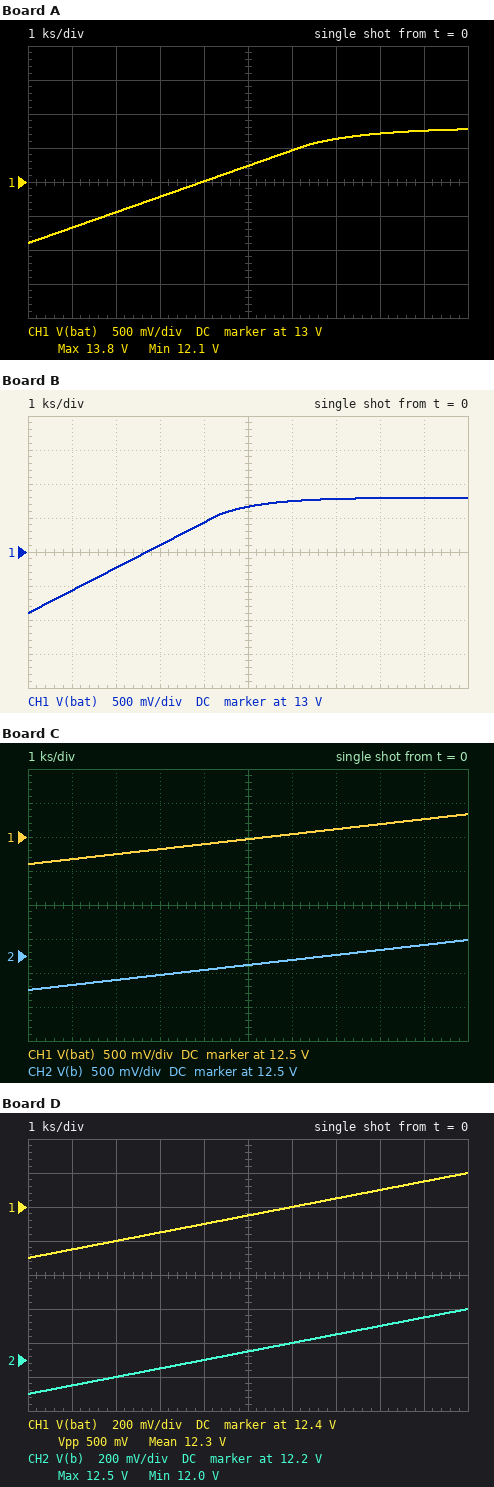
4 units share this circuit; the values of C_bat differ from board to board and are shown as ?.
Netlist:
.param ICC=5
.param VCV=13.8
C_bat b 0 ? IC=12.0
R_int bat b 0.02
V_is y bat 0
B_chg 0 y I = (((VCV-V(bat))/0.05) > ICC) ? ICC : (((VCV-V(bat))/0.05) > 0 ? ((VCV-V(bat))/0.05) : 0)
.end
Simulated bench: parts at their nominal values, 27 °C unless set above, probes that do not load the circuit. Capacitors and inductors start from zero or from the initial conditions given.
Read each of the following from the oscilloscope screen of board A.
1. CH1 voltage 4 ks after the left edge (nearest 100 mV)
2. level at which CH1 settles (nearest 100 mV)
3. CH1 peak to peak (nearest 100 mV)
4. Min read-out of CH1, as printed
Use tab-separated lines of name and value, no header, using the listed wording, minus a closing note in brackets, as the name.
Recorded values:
CH1 voltage 4 ks after the left edge	13.0 V
level at which CH1 settles	13.8 V
CH1 peak to peak	1.7 V
Min read-out of CH1, as printed	12.1 V
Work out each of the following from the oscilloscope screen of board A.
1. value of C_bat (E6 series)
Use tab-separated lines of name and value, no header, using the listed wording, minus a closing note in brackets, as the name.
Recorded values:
value of C_bat	22 kF
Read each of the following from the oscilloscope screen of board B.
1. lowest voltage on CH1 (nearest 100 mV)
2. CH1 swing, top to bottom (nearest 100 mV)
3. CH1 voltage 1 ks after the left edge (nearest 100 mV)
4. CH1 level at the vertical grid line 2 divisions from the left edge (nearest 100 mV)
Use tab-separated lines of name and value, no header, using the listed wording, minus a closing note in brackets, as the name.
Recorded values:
lowest voltage on CH1	12.1 V
CH1 swing, top to bottom	1.7 V
CH1 voltage 1 ks after the left edge	12.4 V
CH1 level at the vertical grid line 2 divisions from the left edge	12.8 V
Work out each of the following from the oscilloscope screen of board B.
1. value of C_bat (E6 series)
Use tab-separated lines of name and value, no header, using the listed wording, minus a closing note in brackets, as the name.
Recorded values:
value of C_bat	15 kF
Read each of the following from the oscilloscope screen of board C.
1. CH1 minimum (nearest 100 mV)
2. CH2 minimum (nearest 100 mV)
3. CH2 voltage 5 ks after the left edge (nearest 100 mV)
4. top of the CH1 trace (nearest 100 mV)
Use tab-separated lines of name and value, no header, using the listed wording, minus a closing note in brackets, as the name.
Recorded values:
CH1 minimum	12.1 V
CH2 minimum	12.0 V
CH2 voltage 5 ks after the left edge	12.4 V
top of the CH1 trace	12.8 V
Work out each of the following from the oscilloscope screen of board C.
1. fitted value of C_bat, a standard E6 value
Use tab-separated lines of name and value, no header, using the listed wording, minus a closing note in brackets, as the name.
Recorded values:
fitted value of C_bat, a standard E6 value	68 kF
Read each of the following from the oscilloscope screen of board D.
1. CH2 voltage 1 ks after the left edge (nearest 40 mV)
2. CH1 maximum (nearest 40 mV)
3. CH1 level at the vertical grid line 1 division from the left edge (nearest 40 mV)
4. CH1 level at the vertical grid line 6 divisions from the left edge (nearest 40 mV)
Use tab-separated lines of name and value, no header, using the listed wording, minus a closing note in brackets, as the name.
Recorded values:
CH2 voltage 1 ks after the left edge	12.04 V
CH1 maximum	12.60 V
CH1 level at the vertical grid line 1 division from the left edge	12.16 V
CH1 level at the vertical grid line 6 divisions from the left edge	12.40 V
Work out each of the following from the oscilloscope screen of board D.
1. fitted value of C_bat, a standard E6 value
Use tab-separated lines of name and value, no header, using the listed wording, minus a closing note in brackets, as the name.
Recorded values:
fitted value of C_bat, a standard E6 value	100 kF
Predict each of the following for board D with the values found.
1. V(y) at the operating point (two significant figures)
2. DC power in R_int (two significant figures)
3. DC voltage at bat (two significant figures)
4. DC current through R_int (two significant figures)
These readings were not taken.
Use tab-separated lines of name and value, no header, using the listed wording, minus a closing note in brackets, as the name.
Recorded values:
V(y) at the operating point	100 mV
DC power in R_int	500 mW
DC voltage at bat	100 mV
DC current through R_int	5.0 A
